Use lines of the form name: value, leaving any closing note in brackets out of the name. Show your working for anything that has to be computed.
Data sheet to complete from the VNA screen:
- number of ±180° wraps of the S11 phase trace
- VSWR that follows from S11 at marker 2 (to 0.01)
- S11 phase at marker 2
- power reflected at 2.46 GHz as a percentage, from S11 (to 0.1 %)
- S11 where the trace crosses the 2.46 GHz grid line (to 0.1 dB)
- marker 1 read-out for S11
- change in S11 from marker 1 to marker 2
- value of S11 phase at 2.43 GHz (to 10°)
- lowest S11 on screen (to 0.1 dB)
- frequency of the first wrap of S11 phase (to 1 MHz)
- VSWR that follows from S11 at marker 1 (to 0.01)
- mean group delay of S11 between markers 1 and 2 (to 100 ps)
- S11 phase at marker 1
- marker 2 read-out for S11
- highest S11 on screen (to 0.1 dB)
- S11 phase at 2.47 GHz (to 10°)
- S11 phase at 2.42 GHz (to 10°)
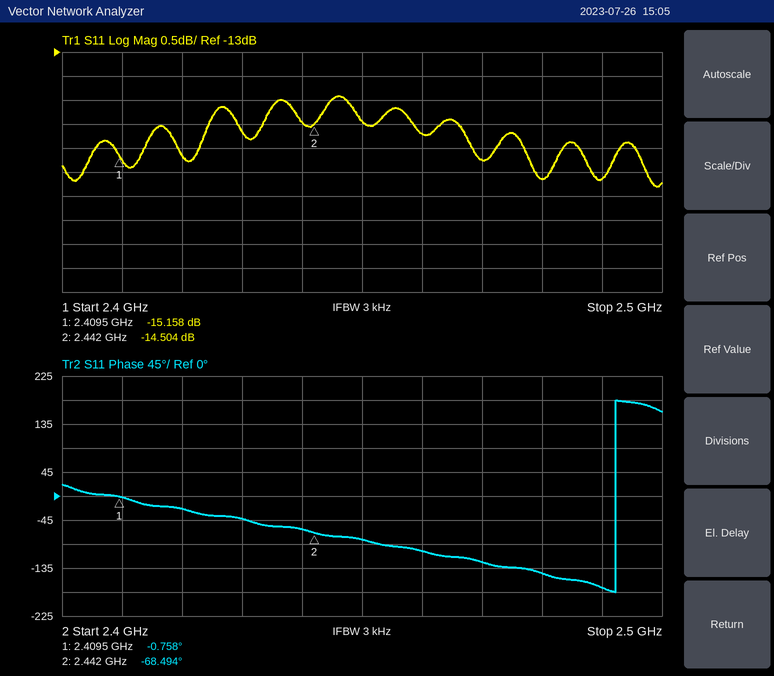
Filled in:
number of ±180° wraps of the S11 phase trace: 1
VSWR that follows from S11 at marker 2: (1 + 0.1883)/(1 − 0.1883) ≈ 1.46
S11 phase at marker 2: -68.494°
power reflected at 2.46 GHz as a percentage, from S11: 10^(-14.7/10) ≈ 3.4 %
S11 where the trace crosses the 2.46 GHz grid line: -14.7 dB
marker 1 read-out for S11: -15.158 dB
change in S11 from marker 1 to marker 2: -14.504 − (-15.158) = 0.654 dB
value of S11 phase at 2.43 GHz: -40°
lowest S11 on screen: -15.8 dB
frequency of the first wrap of S11 phase: 2.492 GHz
VSWR that follows from S11 at marker 1: (1 + 0.1746)/(1 − 0.1746) ≈ 1.42
mean group delay of S11 between markers 1 and 2: −(-68.494° − (-0.758°))/(360° × 32.5 MHz) ≈ 5.8 ns
S11 phase at marker 1: -0.758°
marker 2 read-out for S11: -14.504 dB
highest S11 on screen: -13.9 dB
S11 phase at 2.47 GHz: -120°
S11 phase at 2.42 GHz: -20°
